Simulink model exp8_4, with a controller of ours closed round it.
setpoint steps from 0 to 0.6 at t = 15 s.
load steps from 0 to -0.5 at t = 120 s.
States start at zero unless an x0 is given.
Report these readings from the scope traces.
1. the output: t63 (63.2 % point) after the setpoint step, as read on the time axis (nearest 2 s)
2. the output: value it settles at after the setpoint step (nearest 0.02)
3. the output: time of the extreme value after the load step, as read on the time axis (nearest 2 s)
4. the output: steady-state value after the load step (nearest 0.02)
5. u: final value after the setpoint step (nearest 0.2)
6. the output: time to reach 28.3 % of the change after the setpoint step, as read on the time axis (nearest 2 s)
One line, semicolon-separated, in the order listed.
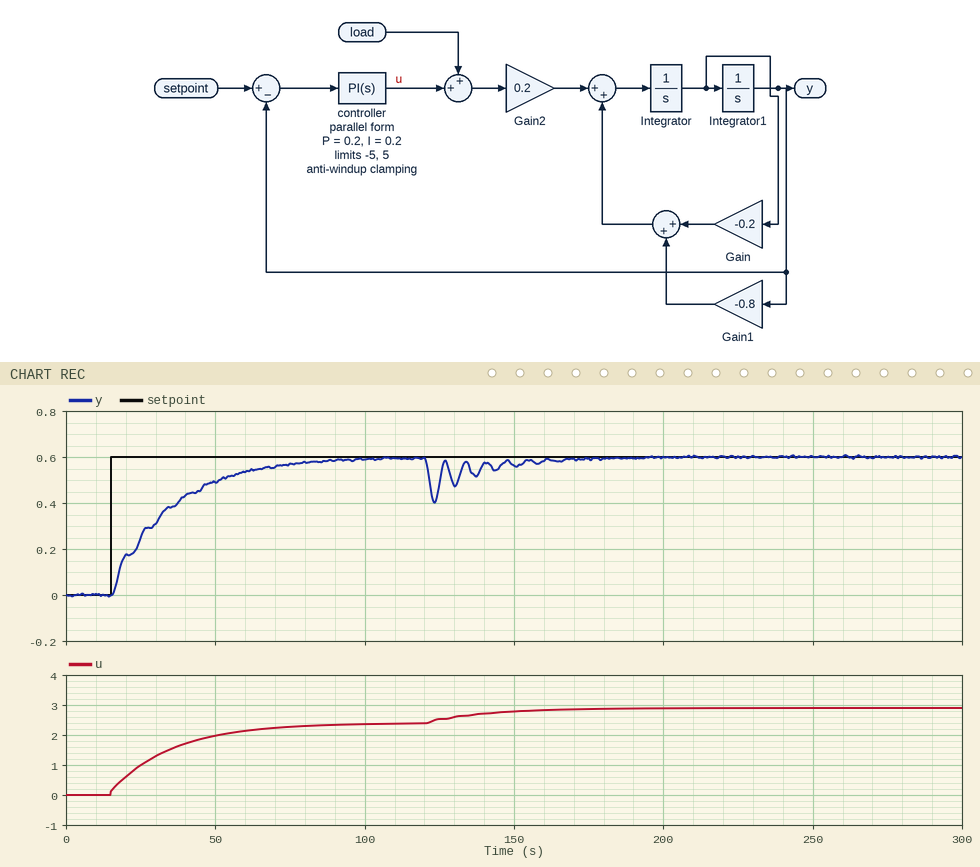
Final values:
34 s; 0.60; 124 s; 0.60; 2.4; 20 s
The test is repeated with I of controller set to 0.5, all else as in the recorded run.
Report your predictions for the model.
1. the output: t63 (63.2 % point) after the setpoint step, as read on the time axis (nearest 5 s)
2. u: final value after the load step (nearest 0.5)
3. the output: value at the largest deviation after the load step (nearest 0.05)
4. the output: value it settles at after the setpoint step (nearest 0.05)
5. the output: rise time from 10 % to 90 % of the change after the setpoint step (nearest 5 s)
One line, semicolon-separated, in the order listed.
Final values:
25 s; 3.0; 0.40; 0.60; 15 s
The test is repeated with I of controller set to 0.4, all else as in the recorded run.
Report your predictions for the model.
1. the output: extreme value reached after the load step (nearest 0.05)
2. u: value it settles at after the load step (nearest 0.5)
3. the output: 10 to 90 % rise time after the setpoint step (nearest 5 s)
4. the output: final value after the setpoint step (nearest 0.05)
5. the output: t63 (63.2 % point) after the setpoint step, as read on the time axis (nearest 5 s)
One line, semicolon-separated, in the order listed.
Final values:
0.40; 3.0; 20 s; 0.60; 25 s
